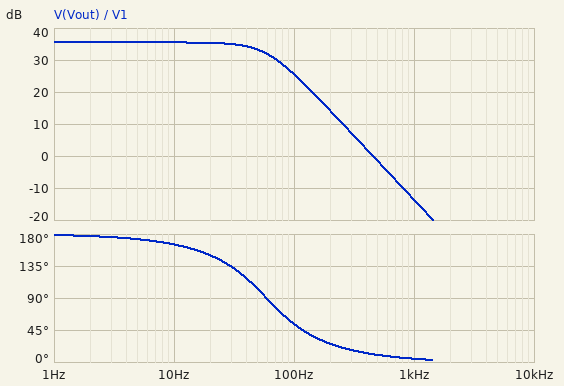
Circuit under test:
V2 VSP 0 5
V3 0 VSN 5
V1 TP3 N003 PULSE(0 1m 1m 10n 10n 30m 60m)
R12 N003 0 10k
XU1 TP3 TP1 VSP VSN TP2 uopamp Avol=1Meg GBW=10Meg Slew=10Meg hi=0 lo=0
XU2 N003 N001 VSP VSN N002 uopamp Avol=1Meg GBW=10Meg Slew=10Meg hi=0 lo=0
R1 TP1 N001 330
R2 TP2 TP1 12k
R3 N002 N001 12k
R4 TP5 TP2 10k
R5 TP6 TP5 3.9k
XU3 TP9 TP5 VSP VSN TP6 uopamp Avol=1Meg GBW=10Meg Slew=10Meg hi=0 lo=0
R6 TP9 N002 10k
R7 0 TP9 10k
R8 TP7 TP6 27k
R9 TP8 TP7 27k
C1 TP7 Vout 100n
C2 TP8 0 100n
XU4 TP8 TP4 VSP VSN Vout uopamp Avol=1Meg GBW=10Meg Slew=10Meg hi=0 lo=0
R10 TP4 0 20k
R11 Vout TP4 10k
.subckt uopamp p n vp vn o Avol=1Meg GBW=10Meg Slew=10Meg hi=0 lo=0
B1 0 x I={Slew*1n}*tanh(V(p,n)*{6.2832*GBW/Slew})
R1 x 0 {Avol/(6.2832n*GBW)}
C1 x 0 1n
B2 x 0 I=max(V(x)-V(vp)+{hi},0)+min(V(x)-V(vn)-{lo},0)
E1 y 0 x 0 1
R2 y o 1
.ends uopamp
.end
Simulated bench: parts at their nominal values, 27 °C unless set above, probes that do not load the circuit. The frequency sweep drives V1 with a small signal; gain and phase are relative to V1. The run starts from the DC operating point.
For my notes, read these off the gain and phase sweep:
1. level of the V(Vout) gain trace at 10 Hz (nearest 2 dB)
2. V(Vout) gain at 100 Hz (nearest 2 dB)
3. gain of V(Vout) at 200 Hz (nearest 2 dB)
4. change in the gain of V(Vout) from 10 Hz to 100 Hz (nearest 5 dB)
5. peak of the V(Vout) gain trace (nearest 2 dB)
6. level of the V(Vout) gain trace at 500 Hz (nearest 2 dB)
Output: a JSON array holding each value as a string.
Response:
["36 dB", "26 dB", "14 dB", "-10 dB", "36 dB", "-2 dB"]
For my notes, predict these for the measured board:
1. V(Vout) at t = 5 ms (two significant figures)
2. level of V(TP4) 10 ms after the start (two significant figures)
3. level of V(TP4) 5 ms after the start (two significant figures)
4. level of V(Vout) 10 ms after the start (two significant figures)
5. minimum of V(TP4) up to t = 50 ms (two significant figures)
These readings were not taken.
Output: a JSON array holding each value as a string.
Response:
["-30 mV", "-39 mV", "-20 mV", "-58 mV", "-41 mV"]
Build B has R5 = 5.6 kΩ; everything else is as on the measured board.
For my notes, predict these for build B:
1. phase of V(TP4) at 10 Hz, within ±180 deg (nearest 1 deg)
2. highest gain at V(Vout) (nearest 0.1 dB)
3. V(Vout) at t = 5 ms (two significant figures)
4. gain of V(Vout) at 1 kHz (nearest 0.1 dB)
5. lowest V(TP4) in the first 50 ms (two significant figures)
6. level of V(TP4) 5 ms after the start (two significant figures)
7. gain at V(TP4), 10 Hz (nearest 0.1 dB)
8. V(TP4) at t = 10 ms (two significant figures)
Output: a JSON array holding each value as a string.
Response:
["165 deg", "37.4 dB", "-37 mV", "-11.8 dB", "-51 mV", "-25 mV", "33.8 dB", "-48 mV"]
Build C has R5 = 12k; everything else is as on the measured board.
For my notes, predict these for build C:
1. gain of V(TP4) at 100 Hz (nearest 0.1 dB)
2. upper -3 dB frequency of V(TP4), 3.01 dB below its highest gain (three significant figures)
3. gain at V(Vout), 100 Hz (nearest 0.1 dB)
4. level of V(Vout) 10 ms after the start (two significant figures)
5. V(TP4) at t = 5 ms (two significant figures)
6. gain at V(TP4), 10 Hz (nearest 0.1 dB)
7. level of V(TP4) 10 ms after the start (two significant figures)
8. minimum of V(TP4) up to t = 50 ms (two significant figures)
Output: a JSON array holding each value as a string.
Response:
["28.6 dB", "55.4 Hz", "32.1 dB", "-120 mV", "-43 mV", "38.5 dB", "-83 mV", "-87 mV"]
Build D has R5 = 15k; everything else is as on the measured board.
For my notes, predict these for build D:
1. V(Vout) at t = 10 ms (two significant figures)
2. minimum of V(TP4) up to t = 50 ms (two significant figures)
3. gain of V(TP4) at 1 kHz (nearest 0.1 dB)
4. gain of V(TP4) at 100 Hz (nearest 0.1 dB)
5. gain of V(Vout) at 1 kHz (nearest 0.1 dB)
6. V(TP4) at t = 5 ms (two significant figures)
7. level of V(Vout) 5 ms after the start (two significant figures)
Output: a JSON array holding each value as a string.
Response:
["-150 mV", "-100 mV", "-9.1 dB", "30.1 dB", "-5.5 dB", "-51 mV", "-77 mV"]
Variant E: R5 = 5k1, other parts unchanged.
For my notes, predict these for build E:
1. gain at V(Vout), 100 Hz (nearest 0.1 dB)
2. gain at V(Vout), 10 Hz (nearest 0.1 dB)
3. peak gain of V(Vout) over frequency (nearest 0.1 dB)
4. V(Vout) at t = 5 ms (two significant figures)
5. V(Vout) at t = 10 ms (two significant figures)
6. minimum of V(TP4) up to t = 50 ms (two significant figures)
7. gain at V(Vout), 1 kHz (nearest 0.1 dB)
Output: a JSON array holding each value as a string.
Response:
["26.9 dB", "36.8 dB", "36.9 dB", "-35 mV", "-68 mV", "-48 mV", "-12.3 dB"]
